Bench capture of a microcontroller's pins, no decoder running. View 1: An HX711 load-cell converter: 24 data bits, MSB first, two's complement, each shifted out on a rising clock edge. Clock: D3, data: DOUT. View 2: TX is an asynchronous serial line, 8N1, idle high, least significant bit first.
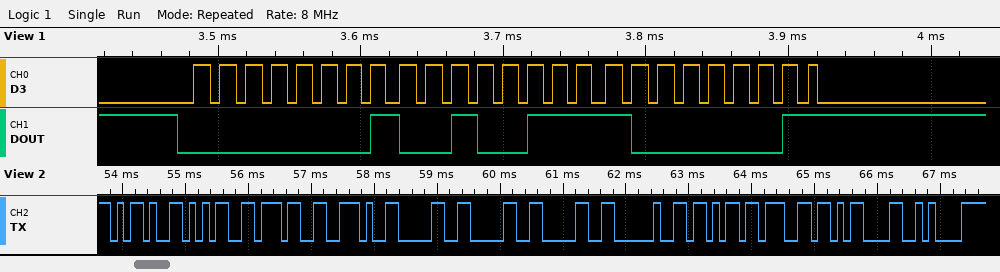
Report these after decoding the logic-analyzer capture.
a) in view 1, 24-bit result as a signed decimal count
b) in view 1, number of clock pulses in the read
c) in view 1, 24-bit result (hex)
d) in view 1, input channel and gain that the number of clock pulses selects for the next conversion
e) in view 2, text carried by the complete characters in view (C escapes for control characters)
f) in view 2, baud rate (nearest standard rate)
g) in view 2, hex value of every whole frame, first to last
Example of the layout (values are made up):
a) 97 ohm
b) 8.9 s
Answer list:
a) 75649
b) 25
c) 0x012781
d) channel A, gain 128
e) "-57.000 kg\r\n"
f) 9600 baud
g) 2D 35 37 2E 30 30 30 20 6B 67 0D 0A
